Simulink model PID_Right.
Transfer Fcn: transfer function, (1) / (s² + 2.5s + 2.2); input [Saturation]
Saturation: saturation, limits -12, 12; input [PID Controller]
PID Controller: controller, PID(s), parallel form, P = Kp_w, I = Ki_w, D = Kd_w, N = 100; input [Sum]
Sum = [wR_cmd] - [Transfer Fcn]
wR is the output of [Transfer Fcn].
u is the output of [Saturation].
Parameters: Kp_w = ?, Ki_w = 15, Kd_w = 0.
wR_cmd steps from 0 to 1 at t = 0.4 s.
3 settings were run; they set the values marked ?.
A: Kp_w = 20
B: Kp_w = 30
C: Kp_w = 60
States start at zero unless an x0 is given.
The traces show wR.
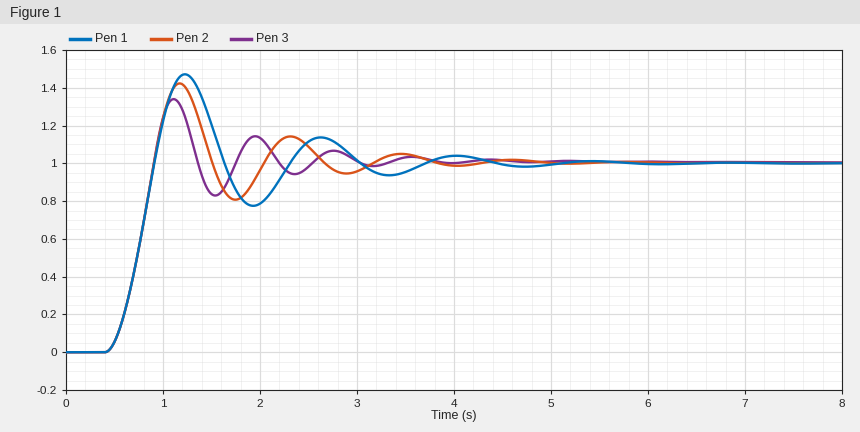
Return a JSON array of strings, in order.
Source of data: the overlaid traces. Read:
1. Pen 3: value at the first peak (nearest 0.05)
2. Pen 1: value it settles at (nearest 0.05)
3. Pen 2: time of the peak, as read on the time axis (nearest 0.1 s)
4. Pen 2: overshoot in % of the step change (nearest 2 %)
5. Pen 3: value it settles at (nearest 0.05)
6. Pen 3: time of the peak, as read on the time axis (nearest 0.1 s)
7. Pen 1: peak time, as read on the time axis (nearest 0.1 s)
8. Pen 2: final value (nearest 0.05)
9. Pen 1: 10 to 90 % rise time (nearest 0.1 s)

["1.35", "1.00", "1.2 s", "42 %", "1.00", "1.1 s", "1.2 s", "1.00", "0.3 s"]
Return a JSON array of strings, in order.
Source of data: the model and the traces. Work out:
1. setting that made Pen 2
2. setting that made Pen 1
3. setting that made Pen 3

["B", "A", "C"]
